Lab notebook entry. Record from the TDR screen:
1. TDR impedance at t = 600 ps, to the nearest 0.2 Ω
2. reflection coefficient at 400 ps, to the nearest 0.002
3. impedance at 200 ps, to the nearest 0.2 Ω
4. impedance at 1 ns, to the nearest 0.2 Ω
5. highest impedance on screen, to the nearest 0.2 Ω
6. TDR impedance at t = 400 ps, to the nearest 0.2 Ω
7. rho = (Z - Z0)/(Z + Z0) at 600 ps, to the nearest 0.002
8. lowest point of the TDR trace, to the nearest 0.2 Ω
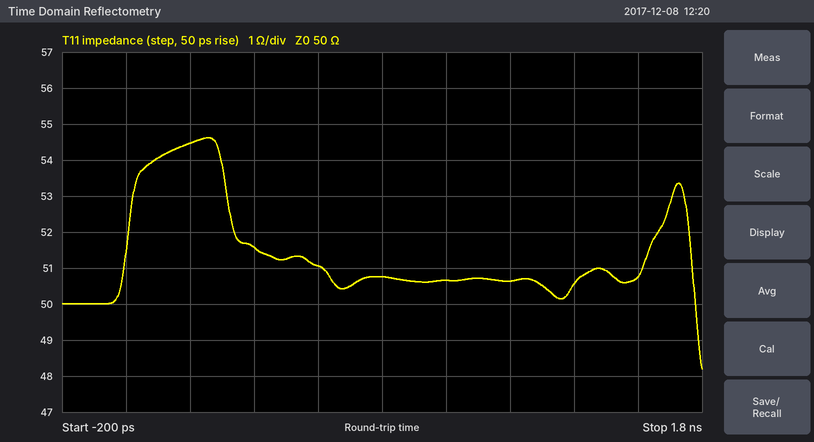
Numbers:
51.0 Ω
+0.016
54.4 Ω
50.6 Ω
54.6 Ω
51.6 Ω
+0.010
48.2 Ω
